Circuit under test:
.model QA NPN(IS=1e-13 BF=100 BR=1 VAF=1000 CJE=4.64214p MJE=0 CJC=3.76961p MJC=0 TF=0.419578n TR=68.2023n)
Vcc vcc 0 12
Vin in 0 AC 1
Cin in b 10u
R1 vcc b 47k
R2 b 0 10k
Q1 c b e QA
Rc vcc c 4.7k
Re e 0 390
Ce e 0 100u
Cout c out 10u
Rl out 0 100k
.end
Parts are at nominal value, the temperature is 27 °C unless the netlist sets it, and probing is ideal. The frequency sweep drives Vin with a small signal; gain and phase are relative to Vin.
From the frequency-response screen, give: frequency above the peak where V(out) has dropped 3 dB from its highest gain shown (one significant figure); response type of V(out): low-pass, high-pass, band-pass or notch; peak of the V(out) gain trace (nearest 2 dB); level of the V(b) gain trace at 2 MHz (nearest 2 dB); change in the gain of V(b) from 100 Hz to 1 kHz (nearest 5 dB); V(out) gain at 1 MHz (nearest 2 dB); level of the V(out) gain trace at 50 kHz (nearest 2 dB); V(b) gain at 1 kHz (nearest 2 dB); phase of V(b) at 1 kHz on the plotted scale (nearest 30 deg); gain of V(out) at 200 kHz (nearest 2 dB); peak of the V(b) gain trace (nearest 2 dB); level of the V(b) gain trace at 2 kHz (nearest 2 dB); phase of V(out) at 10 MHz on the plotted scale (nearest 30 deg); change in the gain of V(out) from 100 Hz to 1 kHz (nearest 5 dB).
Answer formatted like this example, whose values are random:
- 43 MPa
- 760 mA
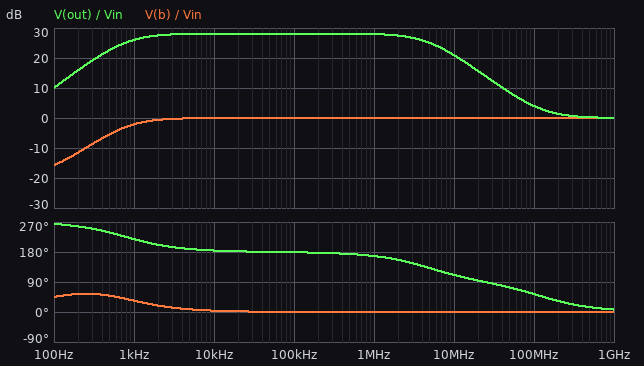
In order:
- 5 MHz
- band-pass
- 28 dB
- 0 dB
- 15 dB
- 28 dB
- 28 dB
- -2 dB
- 30 deg
- 28 dB
- 0 dB
- 0 dB
- 120 deg
- 15 dB
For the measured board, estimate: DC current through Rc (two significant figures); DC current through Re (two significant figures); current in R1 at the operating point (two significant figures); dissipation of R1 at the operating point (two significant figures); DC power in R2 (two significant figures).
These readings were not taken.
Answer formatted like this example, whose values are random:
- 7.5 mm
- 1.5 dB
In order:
- 2.3 mA
- 2.4 mA
- 220 µA
- 2.3 mW
- 240 µW
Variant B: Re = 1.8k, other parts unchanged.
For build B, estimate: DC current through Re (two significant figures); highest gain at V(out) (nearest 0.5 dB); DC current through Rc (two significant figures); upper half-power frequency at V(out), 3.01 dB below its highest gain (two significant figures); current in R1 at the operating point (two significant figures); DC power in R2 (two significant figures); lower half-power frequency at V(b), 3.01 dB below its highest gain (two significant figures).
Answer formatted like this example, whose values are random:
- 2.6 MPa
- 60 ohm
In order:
- 810 µA
- 43.0 dB
- 800 µA
- 9.4 MHz
- 210 µA
- 420 µW
- 2.3 Hz
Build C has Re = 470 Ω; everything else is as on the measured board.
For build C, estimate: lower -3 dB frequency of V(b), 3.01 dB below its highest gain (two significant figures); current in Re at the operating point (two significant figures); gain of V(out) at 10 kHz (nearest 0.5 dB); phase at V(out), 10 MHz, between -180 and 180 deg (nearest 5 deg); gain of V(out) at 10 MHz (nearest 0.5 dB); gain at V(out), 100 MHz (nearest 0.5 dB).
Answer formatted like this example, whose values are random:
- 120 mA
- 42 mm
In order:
- 730 Hz
- 2.3 mA
- 32.5 dB
- 115 deg
- 25.5 dB
- 7.5 dB
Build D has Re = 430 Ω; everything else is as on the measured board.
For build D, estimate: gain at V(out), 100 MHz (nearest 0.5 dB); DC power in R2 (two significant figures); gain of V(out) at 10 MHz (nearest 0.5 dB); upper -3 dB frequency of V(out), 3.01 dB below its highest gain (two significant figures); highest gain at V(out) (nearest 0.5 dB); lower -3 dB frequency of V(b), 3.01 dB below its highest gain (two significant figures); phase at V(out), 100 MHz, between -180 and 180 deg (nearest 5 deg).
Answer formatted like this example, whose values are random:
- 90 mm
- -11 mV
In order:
- 5.5 dB
- 270 µW
- 23.0 dB
- 4.9 MHz
- 30.0 dB
- 760 Hz
- 60 deg
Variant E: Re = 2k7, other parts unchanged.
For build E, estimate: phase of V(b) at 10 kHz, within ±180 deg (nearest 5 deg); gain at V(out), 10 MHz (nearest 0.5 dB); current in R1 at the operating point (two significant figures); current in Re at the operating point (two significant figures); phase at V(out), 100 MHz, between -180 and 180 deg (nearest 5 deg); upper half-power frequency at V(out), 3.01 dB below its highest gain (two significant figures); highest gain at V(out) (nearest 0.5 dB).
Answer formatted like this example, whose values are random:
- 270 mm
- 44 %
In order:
- 0 deg
- 36.0 dB
- 210 µA
- 550 µA
- 90 deg
- 9.4 MHz
- 39.5 dB
